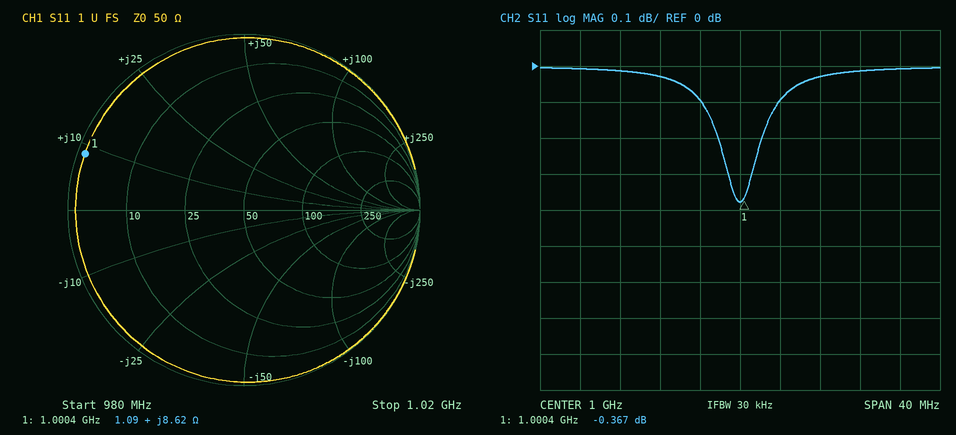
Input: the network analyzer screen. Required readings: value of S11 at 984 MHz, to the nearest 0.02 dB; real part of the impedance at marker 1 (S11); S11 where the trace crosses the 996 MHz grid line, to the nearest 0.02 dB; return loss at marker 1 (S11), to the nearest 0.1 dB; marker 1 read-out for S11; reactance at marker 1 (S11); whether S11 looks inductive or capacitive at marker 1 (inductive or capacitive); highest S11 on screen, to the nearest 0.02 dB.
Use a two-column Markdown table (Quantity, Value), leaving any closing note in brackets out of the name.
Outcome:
| Quantity | Value |
|---|---|
| value of S11 at 984 MHz, to the nearest 0.02 dB | 0.00 dB |
| real part of the impedance at marker 1 | 1.09 Ω |
| S11 where the trace crosses the 996 MHz grid line, to the nearest 0.02 dB | -0.10 dB |
| return loss at marker 1 (S11), to the nearest 0.1 dB | 0.4 dB |
| marker 1 read-out for S11 | -0.367 dB |
| reactance at marker 1 | +8.62 Ω |
| whether S11 looks inductive or capacitive at marker 1 | inductive |
| highest S11 on screen, to the nearest 0.02 dB | 0.00 dB |
